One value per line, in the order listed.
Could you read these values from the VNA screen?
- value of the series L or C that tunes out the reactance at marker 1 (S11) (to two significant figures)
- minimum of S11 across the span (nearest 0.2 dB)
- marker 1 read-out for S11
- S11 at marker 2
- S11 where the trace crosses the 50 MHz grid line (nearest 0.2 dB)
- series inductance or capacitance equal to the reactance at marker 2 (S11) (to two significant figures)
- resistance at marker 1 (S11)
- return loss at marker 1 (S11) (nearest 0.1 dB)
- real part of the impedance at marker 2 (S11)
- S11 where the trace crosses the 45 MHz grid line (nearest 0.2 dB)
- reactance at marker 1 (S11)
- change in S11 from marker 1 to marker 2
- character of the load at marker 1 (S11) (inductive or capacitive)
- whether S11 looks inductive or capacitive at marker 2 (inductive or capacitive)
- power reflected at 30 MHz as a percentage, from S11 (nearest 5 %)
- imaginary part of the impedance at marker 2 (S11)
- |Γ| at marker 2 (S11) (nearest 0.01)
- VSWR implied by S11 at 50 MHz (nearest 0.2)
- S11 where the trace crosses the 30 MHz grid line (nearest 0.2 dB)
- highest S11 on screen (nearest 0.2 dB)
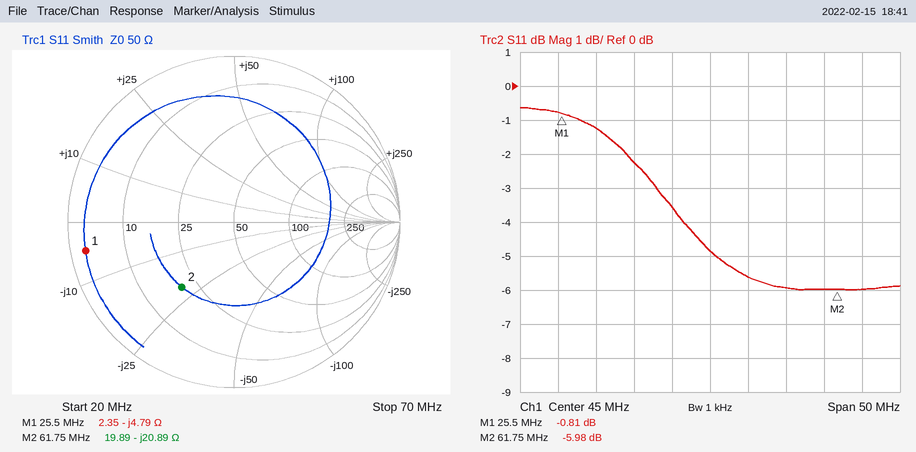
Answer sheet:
30 nH
-6.0 dB
-0.81 dB
-5.98 dB
-5.6 dB
120 pF
2.35 Ω
0.8 dB
19.89 Ω
-4.8 dB
-4.79 Ω
-5.17 dB
capacitive
capacitive
75 %
-20.89 Ω
0.50
3.2
-1.2 dB
-0.6 dB
